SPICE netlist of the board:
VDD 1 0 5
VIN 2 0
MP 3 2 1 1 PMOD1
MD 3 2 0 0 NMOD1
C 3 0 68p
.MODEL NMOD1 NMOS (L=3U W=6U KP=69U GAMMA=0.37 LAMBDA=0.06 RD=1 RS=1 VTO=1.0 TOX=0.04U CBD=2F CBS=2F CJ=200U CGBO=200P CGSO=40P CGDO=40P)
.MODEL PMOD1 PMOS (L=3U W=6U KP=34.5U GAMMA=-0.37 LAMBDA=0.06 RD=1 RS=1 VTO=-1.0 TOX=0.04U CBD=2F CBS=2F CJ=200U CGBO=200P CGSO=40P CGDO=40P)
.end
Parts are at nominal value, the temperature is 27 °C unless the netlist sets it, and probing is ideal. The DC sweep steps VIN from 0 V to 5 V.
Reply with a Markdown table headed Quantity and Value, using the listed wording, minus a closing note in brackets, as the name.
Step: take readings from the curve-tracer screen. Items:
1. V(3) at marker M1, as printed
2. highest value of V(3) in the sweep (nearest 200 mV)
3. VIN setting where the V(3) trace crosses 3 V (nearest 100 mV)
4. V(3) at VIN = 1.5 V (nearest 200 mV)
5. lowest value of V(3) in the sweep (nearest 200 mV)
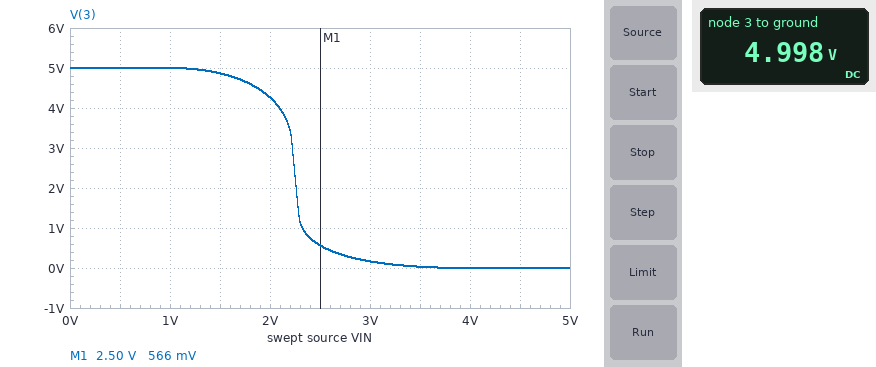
| Quantity | Value |
|---|---|
| V(3) at marker M1, as printed | 566 mV |
| highest value of V(3) in the sweep | 5.0 V |
| VIN setting where the V(3) trace crosses 3 V | 2.2 V |
| V(3) at VIN = 1.5 V | 4.8 V |
| lowest value of V(3) in the sweep | 0 V |
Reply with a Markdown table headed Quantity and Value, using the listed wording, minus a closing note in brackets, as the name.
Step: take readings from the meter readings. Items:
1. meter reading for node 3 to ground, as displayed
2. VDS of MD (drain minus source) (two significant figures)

| Quantity | Value |
|---|---|
| meter reading for node 3 to ground, as displayed | 4.998 V |
| VDS of MD (drain minus source) | 5.0 V |
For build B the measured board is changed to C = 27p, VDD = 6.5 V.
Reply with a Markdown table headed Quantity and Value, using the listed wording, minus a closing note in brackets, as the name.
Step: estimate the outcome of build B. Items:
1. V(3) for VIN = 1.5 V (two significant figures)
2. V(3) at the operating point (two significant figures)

| Quantity | Value |
|---|---|
| V(3) for VIN = 1.5 V | 6.4 V |
| V(3) at the operating point | 6.5 V |
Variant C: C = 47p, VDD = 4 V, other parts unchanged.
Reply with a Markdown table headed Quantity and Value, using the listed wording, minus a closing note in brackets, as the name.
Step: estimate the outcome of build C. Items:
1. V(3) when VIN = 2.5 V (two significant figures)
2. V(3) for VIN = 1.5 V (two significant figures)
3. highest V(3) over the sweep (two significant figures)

| Quantity | Value |
|---|---|
| V(3) when VIN = 2.5 V | 52 mV |
| V(3) for VIN = 1.5 V | 3.8 V |
| highest V(3) over the sweep | 4.0 V |
